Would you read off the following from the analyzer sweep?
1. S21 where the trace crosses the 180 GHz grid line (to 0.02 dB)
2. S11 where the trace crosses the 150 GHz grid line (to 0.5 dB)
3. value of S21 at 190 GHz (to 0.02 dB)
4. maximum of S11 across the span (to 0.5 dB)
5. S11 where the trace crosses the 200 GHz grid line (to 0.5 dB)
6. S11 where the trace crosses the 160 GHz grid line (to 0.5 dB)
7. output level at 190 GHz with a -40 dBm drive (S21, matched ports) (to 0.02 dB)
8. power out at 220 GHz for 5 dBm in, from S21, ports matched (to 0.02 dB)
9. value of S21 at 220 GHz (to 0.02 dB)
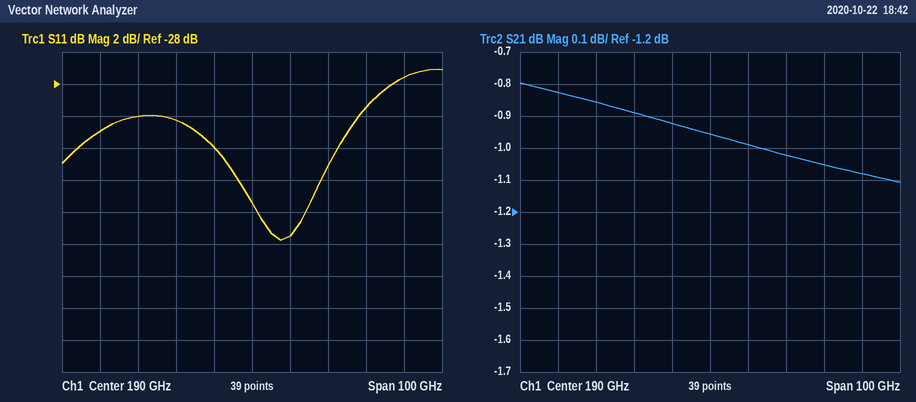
-0.92 dB
-31.0 dB
-0.96 dB
-27.0 dB
-37.5 dB
-30.0 dB
-40.96 dBm
3.94 dBm
-1.06 dB
